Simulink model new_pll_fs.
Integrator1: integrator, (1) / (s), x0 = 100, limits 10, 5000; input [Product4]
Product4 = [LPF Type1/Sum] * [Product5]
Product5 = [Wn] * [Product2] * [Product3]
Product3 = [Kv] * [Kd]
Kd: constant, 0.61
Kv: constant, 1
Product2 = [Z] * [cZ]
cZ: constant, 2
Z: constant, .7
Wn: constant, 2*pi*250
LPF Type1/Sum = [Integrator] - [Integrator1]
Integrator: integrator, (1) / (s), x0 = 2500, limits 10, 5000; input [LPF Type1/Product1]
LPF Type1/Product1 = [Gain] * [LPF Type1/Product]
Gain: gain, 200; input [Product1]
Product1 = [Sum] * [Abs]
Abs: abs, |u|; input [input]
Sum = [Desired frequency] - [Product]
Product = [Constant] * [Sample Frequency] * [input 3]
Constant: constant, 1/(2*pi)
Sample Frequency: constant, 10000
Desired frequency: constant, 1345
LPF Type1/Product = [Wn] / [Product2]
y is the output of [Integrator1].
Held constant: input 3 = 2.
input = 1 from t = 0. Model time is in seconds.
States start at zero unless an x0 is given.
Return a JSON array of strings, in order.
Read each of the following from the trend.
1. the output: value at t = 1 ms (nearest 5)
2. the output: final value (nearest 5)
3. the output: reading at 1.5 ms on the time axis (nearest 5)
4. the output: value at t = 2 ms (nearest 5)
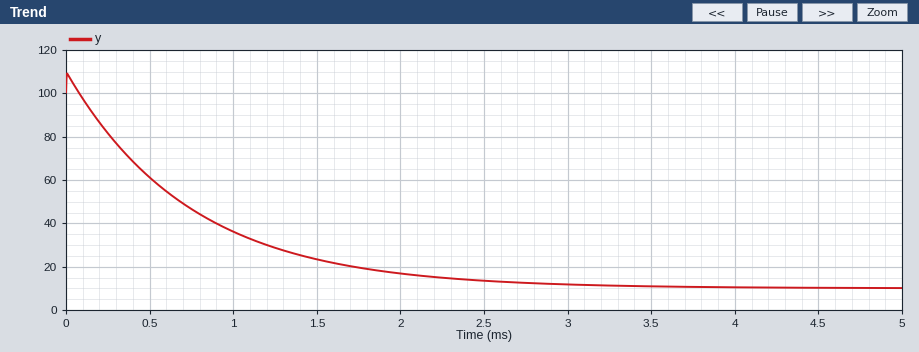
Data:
["35", "10", "25", "15"]
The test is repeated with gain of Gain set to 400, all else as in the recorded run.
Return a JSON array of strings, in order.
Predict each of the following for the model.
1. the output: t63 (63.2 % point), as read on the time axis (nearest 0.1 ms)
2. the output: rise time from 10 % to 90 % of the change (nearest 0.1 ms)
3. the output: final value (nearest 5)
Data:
["0.8 ms", "1.6 ms", "10"]
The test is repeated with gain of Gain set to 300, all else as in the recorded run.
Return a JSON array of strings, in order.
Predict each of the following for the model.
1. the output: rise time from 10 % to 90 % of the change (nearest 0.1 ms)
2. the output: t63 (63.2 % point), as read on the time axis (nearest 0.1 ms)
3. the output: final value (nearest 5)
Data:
["1.6 ms", "0.8 ms", "10"]
